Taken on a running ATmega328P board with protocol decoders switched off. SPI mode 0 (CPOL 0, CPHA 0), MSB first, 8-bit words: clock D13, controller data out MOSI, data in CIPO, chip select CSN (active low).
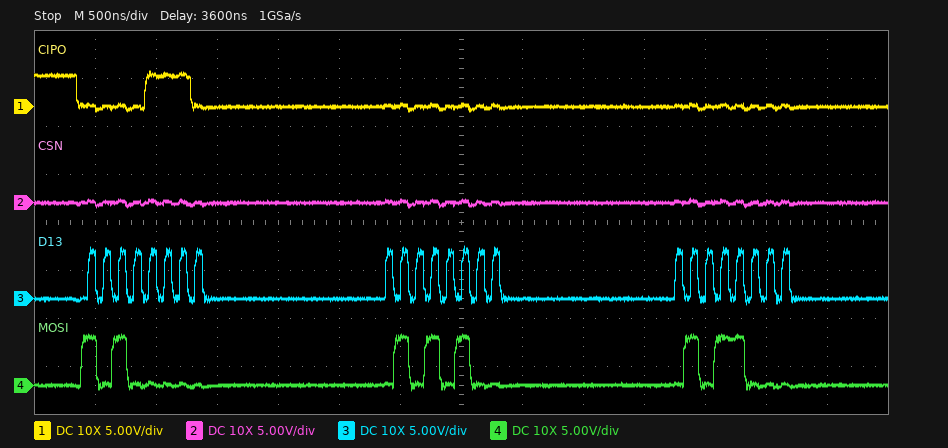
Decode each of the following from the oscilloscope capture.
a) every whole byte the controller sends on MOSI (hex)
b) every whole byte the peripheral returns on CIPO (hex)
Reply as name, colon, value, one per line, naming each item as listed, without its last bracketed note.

every whole byte the controller sends on MOSI: A0 54 58
every whole byte the peripheral returns on CIPO: 0E 00 00
